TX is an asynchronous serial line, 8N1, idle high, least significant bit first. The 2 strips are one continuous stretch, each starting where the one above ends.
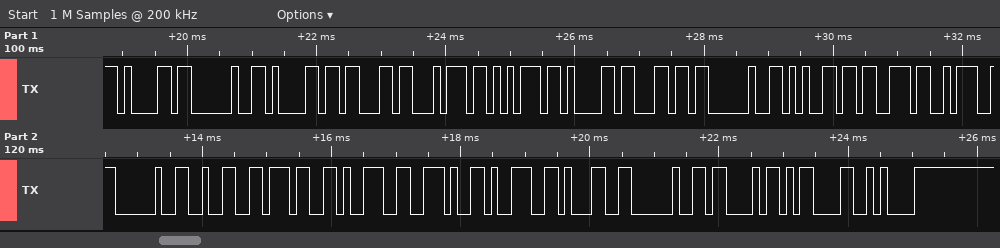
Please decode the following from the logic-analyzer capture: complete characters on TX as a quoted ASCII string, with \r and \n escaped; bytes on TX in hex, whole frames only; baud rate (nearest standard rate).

"a actual es: 279.91 C\r\n"
61 20 61 63 74 75 61 6C 20 65 73 3A 20 32 37 39 2E 39 31 20 43 0D 0A
9600 baud
